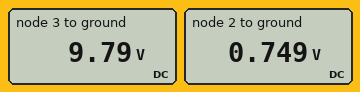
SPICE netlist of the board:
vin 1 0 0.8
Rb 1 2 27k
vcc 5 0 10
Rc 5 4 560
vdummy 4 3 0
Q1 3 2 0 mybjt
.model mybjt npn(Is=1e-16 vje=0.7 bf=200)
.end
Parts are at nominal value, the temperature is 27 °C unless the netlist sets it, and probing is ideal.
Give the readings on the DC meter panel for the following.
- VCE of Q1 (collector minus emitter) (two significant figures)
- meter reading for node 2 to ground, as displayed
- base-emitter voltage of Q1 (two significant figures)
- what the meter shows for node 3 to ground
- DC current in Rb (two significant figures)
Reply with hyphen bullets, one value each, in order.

- 9.8 V
- 0.749 V
- 750 mV
- 9.79 V
- 1.9 µA
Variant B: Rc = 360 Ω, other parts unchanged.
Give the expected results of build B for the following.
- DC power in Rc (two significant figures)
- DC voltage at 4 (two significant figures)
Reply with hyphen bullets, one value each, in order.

- 51 µW
- 9.9 V
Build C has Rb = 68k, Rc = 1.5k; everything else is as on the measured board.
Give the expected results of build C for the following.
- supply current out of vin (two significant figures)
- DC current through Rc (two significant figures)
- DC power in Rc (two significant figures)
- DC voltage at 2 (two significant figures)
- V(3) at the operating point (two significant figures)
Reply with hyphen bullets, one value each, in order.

- 990 nA
- 200 µA
- 59 µW
- 730 mV
- 9.7 V
